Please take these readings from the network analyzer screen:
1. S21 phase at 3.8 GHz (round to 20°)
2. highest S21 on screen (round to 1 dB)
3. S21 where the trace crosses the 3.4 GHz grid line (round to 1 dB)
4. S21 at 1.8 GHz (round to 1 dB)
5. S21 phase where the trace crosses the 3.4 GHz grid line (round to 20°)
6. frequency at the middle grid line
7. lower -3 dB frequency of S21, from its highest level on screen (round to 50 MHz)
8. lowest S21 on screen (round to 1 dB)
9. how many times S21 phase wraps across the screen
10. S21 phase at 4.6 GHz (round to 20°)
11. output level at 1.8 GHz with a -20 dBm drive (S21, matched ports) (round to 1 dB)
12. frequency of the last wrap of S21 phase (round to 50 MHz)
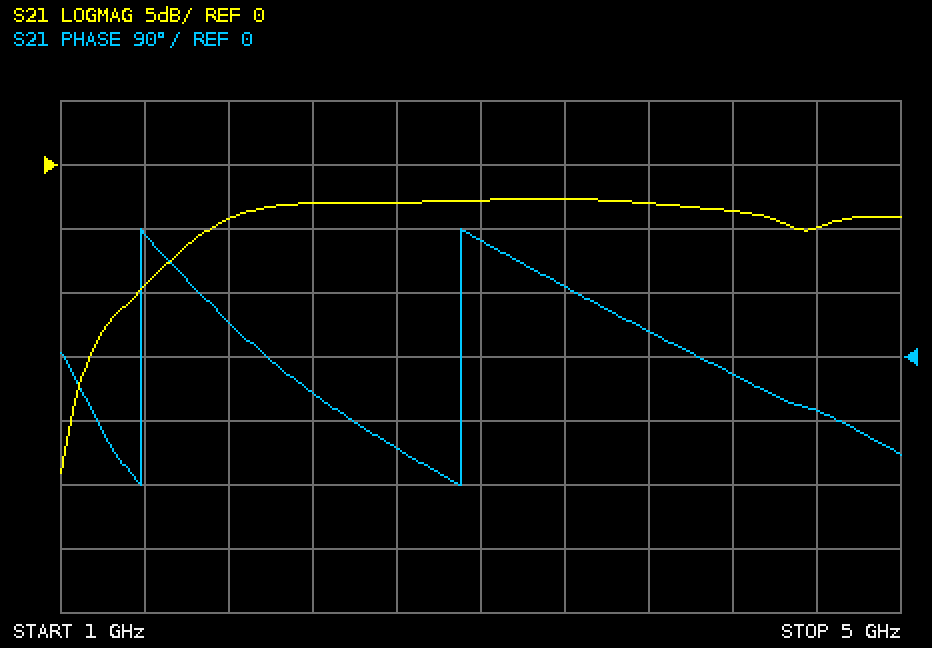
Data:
40°
-3 dB
-3 dB
-4 dB
100°
3 GHz
1.65 GHz
-24 dB
2
-80°
-24 dBm
2.90 GHz
